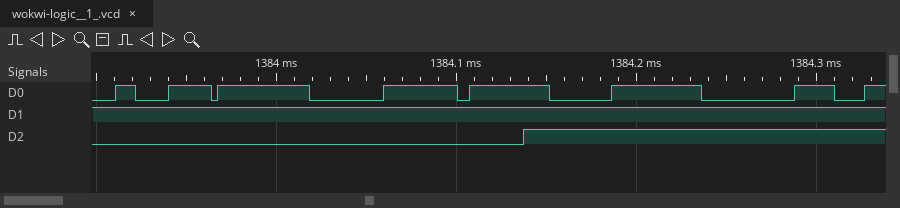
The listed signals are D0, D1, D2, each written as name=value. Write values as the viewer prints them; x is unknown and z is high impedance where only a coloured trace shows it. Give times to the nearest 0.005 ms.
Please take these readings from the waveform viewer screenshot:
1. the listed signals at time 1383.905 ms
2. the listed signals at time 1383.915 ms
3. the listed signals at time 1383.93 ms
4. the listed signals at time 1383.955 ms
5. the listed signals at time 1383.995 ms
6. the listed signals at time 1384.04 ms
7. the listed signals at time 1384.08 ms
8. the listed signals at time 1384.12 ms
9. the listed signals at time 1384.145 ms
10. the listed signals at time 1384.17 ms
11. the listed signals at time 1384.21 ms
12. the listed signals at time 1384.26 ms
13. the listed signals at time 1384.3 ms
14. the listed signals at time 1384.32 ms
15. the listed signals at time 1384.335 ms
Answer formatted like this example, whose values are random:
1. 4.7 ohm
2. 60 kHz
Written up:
1. D0=0, D1=1, D2=0
2. D0=1, D1=1, D2=0
3. D0=0, D1=1, D2=0
4. D0=1, D1=1, D2=0
5. D0=1, D1=1, D2=0
6. D0=0, D1=1, D2=0
7. D0=1, D1=1, D2=0
8. D0=1, D1=1, D2=0
9. D0=1, D1=1, D2=1
10. D0=0, D1=1, D2=1
11. D0=1, D1=1, D2=1
12. D0=0, D1=1, D2=1
13. D0=1, D1=1, D2=1
14. D0=0, D1=1, D2=1
15. D0=1, D1=1, D2=1
